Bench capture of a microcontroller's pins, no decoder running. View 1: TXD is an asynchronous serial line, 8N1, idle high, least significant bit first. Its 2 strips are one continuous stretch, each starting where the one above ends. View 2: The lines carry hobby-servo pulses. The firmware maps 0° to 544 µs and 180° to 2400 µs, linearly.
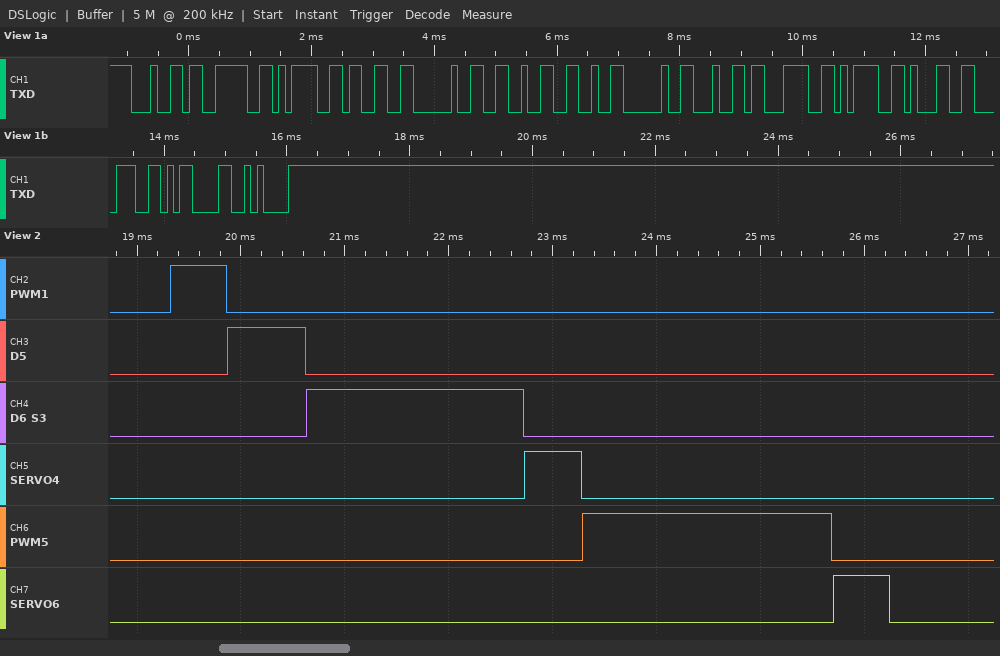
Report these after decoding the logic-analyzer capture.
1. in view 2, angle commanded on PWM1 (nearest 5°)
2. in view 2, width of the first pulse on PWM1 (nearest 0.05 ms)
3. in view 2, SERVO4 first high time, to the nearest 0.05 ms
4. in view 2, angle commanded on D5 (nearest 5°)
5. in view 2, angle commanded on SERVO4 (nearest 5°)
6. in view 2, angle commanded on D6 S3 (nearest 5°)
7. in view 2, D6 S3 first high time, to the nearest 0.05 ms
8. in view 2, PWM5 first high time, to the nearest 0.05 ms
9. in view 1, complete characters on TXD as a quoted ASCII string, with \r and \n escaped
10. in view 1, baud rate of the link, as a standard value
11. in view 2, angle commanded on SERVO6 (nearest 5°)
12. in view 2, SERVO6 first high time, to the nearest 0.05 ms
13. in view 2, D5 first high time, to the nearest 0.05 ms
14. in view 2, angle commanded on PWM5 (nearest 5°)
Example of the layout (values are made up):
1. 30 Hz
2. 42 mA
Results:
1. 0°
2. 0.55 ms
3. 0.55 ms
4. 20°
5. 0°
6. 150°
7. 2.10 ms
8. 2.40 ms
9. "d>=3 && d<=18\r\n"
10. 9600 baud
11. 0°
12. 0.55 ms
13. 0.75 ms
14. 180°
